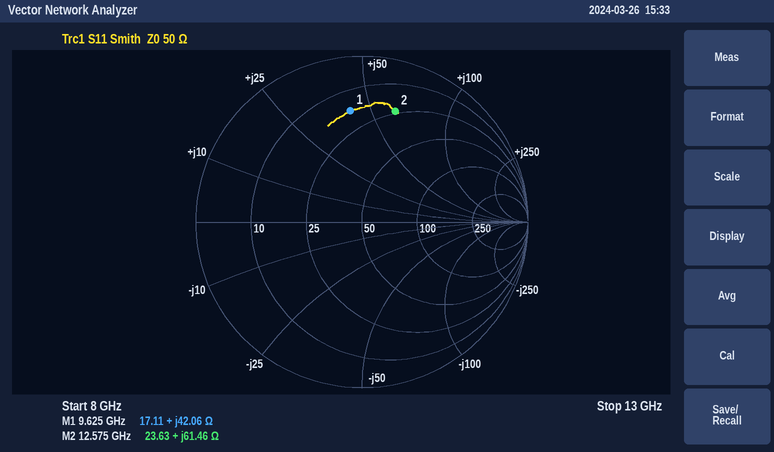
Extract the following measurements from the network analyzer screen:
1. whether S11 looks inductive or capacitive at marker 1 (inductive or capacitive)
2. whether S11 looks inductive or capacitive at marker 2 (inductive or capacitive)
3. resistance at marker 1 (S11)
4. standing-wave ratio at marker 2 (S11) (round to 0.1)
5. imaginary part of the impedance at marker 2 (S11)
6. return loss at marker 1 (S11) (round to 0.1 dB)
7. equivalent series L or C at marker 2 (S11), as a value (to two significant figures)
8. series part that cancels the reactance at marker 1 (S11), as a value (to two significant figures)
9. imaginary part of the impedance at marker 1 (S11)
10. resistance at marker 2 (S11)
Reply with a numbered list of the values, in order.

1. inductive
2. inductive
3. 17.11 Ω
4. 5.6
5. +61.46 Ω
6. 3.4 dB
7. 780 pH
8. 390 fF
9. +42.06 Ω
10. 23.63 Ω
